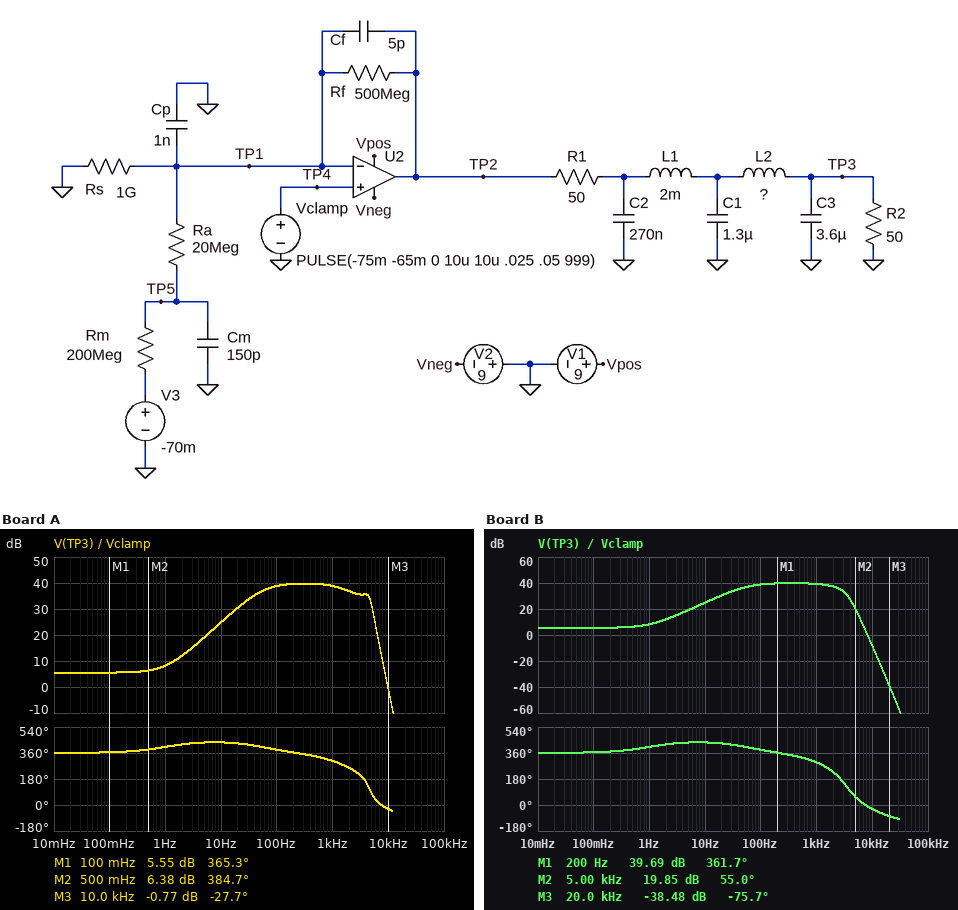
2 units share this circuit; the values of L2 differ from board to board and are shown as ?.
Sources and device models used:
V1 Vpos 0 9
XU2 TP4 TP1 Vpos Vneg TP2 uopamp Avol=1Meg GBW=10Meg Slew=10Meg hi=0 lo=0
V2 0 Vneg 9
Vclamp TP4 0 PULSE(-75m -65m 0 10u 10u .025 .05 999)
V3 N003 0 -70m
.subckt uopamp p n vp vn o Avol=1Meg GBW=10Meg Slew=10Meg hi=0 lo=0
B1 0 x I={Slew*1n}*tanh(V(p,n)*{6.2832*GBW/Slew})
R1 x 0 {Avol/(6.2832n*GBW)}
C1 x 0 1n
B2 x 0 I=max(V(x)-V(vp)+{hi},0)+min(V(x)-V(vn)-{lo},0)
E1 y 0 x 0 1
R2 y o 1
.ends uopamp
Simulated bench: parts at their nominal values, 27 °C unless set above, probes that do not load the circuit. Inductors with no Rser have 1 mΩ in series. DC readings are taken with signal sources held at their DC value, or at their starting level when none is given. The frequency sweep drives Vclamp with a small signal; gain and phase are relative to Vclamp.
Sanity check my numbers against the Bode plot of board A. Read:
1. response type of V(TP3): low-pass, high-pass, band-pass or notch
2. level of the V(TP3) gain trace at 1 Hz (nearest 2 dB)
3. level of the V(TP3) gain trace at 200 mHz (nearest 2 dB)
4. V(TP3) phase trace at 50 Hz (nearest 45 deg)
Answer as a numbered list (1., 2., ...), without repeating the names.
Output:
1. band-pass
2. 8 dB
3. 6 dB
4. 405 deg
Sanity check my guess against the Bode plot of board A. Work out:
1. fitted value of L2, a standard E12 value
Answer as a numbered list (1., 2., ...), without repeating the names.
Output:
1. 1.8 mH
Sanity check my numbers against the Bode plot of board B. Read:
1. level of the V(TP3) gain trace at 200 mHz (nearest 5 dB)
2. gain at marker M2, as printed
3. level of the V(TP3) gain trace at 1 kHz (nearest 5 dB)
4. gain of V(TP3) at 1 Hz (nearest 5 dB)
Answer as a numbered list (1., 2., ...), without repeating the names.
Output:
1. 5 dB
2. 19.85 dB
3. 40 dB
4. 10 dB
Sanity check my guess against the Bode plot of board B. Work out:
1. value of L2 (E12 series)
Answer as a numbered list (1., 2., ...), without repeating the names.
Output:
1. 3.9 mH
